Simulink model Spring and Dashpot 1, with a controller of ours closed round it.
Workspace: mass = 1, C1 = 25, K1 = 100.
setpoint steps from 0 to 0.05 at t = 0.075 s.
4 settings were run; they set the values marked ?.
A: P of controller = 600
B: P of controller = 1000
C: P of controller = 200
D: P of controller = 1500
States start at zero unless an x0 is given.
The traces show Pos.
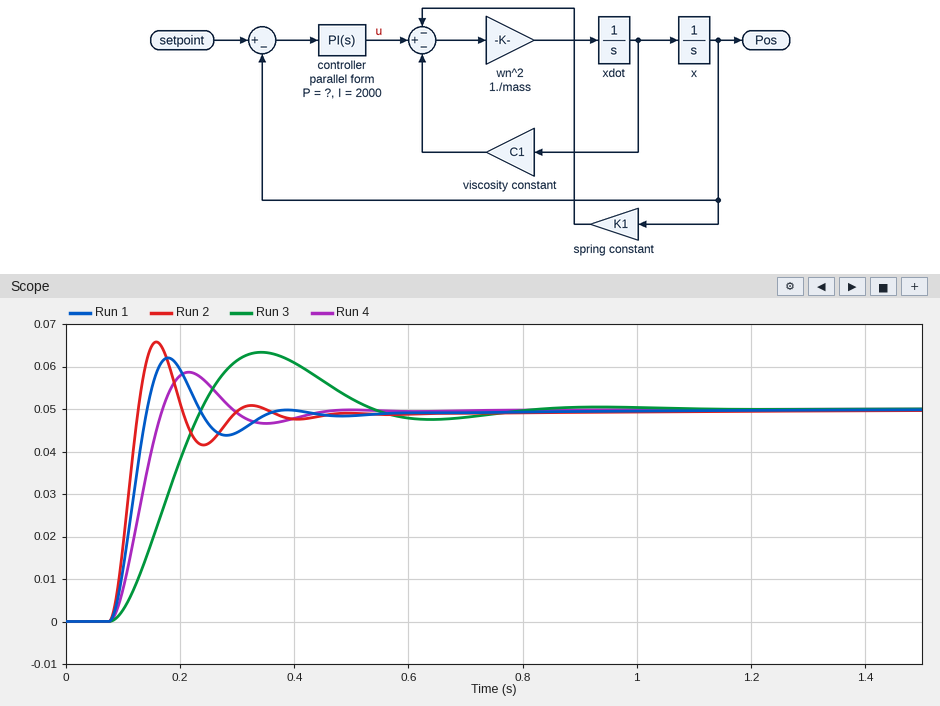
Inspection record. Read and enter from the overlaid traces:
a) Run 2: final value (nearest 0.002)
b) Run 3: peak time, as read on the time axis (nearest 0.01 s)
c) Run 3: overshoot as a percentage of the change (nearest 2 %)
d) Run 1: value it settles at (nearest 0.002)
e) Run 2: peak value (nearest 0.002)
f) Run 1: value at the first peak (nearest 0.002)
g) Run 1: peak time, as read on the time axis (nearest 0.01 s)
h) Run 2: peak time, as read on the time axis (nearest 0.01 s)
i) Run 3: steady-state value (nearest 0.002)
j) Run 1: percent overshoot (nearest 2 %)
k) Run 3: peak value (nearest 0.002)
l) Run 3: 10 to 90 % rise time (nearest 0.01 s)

0.050
0.34 s
26 %
0.050
0.066
0.062
0.18 s
0.16 s
0.050
24 %
0.064
0.11 s
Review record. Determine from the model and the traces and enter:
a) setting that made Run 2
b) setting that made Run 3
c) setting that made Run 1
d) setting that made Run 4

D
C
B
A
